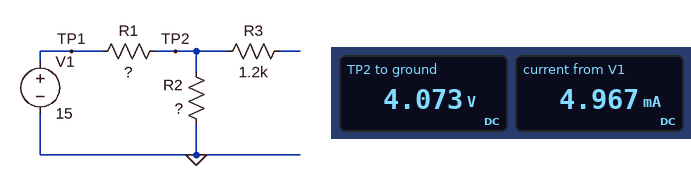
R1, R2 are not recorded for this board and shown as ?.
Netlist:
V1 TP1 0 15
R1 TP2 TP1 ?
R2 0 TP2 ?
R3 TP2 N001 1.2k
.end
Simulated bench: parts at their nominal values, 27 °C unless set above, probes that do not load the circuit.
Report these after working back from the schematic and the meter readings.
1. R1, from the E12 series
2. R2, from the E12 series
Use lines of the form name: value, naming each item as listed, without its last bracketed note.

R1, from the E12 series: 2.2 kΩ
R2, from the E12 series: 820 Ω
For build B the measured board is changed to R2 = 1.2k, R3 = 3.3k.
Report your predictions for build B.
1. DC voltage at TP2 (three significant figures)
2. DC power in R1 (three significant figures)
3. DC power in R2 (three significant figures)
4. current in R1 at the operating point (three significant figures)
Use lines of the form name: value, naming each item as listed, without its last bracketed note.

DC voltage at TP2: 5.29 V
DC power in R1: 42.8 mW
DC power in R2: 23.4 mW
current in R1 at the operating point: 4.41 mA
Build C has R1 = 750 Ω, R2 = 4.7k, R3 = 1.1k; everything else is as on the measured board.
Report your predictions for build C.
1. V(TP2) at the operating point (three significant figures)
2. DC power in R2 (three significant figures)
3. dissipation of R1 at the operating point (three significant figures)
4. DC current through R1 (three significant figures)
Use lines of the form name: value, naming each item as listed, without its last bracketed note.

V(TP2) at the operating point: 12.9 V
DC power in R2: 35.6 mW
dissipation of R1 at the operating point: 5.68 mW
DC current through R1: 2.75 mA
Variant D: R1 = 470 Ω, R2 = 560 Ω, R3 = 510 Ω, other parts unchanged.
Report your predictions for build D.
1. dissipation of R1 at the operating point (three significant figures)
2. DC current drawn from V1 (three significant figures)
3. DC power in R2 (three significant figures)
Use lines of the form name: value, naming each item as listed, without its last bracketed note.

dissipation of R1 at the operating point: 99.7 mW
DC current drawn from V1: 14.6 mA
DC power in R2: 119 mW
